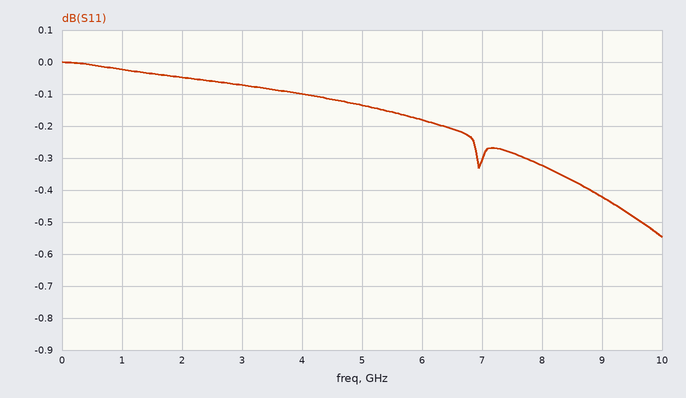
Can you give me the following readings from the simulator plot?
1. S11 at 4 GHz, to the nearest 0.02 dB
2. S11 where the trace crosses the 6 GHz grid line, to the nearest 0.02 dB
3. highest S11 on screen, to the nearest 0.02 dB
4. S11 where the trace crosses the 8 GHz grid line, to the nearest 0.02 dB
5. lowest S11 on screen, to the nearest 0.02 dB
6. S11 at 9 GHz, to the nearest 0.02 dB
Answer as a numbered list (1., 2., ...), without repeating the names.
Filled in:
1. -0.10 dB
2. -0.18 dB
3. 0.00 dB
4. -0.32 dB
5. -0.54 dB
6. -0.42 dB
